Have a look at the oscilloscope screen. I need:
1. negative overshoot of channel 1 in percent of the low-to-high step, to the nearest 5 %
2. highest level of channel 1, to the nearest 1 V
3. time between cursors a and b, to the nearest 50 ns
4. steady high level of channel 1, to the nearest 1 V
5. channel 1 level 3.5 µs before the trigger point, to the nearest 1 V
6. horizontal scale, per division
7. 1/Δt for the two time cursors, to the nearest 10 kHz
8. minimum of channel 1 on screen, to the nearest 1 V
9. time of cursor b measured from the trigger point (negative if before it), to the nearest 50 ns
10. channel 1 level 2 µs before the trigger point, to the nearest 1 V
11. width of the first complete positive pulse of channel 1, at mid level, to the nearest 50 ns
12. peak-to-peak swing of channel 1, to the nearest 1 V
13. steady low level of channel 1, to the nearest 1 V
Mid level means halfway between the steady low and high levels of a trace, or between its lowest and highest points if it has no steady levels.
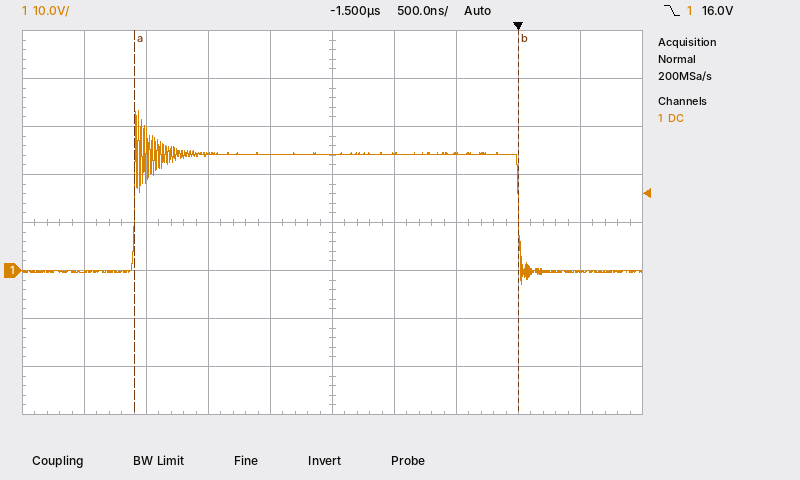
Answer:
10 %
33 V
3.10 µs
24 V
0 V
500 ns
320 kHz
-3 V
0 ns
24 V
3.10 µs
36 V
0 V
